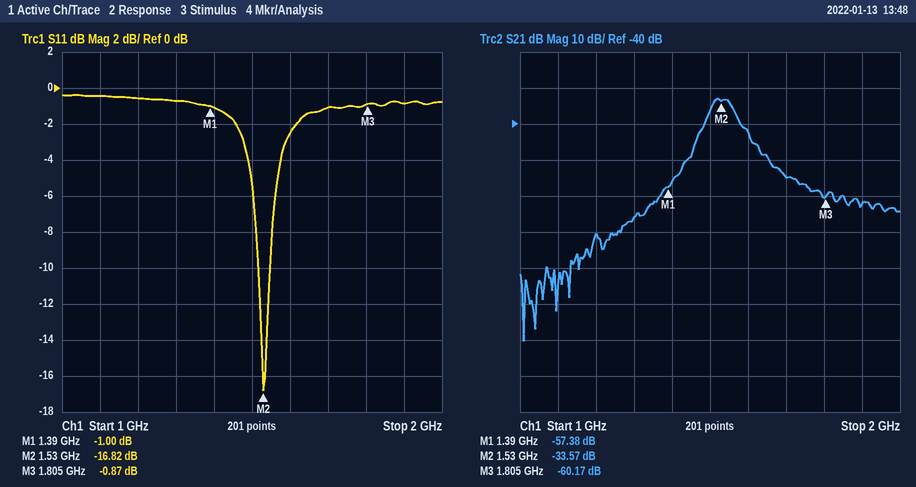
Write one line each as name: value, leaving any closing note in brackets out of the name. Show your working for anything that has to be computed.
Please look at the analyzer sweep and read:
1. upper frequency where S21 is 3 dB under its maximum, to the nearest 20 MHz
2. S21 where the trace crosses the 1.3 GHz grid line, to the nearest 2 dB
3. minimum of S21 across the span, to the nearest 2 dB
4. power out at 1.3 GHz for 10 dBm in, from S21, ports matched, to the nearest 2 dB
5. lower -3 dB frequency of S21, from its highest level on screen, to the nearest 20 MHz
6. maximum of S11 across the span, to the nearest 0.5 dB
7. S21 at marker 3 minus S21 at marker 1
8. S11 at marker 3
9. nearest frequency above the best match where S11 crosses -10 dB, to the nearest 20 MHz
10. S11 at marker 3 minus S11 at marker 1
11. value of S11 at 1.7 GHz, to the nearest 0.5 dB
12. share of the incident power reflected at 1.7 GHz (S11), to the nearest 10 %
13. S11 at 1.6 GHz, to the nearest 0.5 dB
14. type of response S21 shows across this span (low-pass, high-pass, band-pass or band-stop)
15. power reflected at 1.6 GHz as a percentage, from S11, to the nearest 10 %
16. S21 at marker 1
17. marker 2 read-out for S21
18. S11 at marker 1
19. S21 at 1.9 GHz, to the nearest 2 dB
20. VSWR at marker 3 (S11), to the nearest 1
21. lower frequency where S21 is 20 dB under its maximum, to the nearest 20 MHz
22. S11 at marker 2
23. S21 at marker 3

upper frequency where S21 is 3 dB under its maximum, to the nearest 20 MHz: 1.56 GHz
S21 where the trace crosses the 1.3 GHz grid line, to the nearest 2 dB: -66 dB
minimum of S21 across the span, to the nearest 2 dB: -100 dB
power out at 1.3 GHz for 10 dBm in, from S21, ports matched, to the nearest 2 dB: 10 dBm + (-66 dB) = -56 dBm
lower -3 dB frequency of S21, from its highest level on screen, to the nearest 20 MHz: 1.50 GHz
maximum of S11 across the span, to the nearest 0.5 dB: -0.5 dB
S21 at marker 3 minus S21 at marker 1: -60.17 − (-57.38) = -2.79 dB
S11 at marker 3: -0.87 dB
nearest frequency above the best match where S11 crosses -10 dB, to the nearest 20 MHz: 1.54 GHz
S11 at marker 3 minus S11 at marker 1: -0.87 − (-1) = 0.13 dB
value of S11 at 1.7 GHz, to the nearest 0.5 dB: -1.0 dB
share of the incident power reflected at 1.7 GHz (S11), to the nearest 10 %: 10^(-1/10) ≈ 79.4 %, so 80 % to the nearest 10 %
S11 at 1.6 GHz, to the nearest 0.5 dB: -2.5 dB
type of response S21 shows across this span: band-pass
power reflected at 1.6 GHz as a percentage, from S11, to the nearest 10 %: 10^(-2.5/10) ≈ 56.2 %, so 60 % to the nearest 10 %
S21 at marker 1: -57.38 dB
marker 2 read-out for S21: -33.57 dB
S11 at marker 1: -1.00 dB
S21 at 1.9 GHz, to the nearest 2 dB: -62 dB
VSWR at marker 3 (S11), to the nearest 1: (1 + 0.9047)/(1 − 0.9047) ≈ 20
lower frequency where S21 is 20 dB under its maximum, to the nearest 20 MHz: 1.42 GHz
S11 at marker 2: -16.82 dB
S21 at marker 3: -60.17 dB
